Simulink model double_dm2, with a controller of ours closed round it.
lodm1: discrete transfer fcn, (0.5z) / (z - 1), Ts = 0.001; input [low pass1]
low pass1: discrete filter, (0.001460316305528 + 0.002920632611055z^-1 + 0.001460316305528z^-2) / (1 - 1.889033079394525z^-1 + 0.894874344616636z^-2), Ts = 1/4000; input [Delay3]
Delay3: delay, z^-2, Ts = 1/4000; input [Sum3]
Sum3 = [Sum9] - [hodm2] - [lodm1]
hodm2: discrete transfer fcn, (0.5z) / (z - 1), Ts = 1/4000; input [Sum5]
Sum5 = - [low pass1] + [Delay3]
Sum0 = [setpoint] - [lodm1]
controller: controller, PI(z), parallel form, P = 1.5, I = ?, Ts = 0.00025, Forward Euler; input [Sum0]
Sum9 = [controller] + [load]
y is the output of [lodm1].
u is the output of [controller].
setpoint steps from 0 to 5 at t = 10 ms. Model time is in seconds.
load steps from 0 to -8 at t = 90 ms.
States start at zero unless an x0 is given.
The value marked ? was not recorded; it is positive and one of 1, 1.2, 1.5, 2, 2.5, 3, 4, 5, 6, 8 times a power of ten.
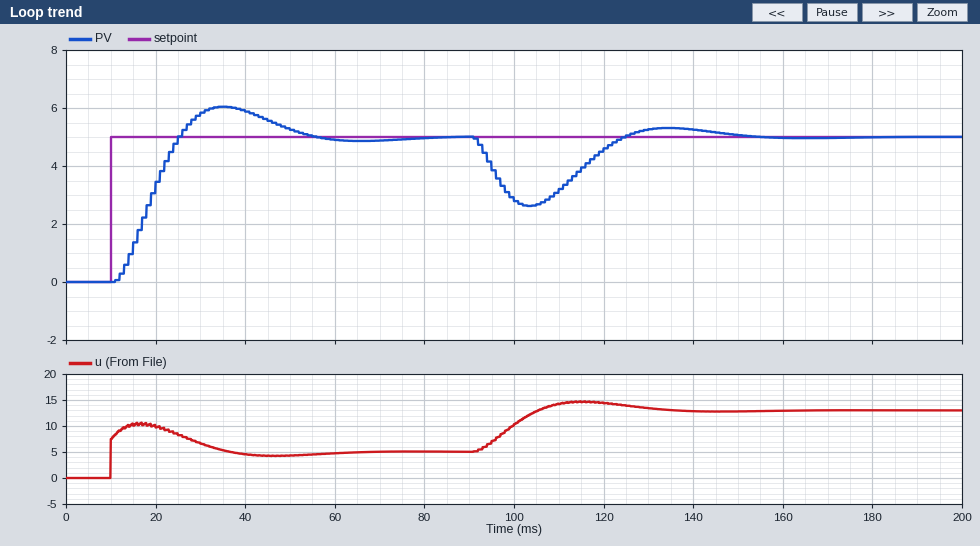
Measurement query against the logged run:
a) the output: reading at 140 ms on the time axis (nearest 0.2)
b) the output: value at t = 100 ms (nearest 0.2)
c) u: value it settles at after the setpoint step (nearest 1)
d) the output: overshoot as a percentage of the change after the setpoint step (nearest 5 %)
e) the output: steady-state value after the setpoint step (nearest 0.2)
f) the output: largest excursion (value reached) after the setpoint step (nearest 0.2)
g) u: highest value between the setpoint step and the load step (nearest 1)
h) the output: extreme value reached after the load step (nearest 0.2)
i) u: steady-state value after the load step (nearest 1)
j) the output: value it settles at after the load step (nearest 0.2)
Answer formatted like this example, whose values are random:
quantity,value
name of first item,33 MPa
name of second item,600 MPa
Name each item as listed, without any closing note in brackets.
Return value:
quantity,value
the output: reading at 140 ms on the time axis,5.2
the output: value at t = 100 ms,2.8
u: value it settles at after the setpoint step,5
the output: overshoot as a percentage of the change after the setpoint step,20 %
the output: steady-state value after the setpoint step,5.0
the output: largest excursion (value reached) after the setpoint step,6.0
u: highest value between the setpoint step and the load step,11
the output: extreme value reached after the load step,2.6
u: steady-state value after the load step,13
the output: value it settles at after the load step,5.0
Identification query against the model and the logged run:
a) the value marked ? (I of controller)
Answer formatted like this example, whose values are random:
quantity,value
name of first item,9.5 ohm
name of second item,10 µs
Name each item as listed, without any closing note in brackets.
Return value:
quantity,value
the value marked ?,200
